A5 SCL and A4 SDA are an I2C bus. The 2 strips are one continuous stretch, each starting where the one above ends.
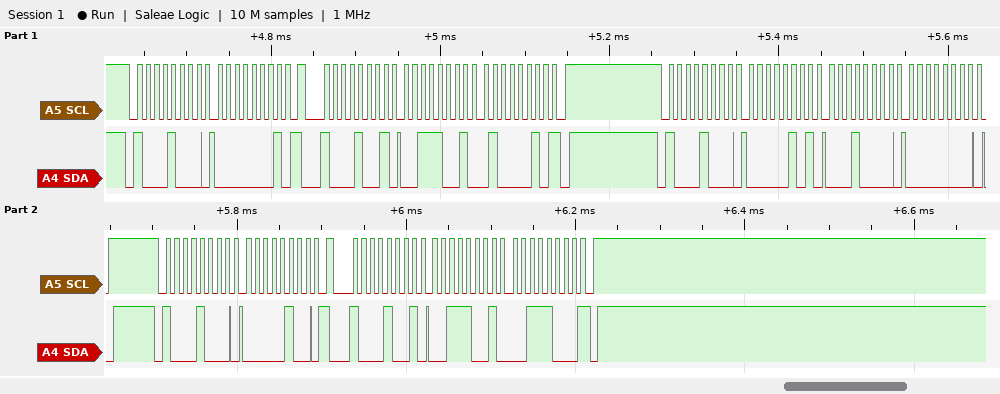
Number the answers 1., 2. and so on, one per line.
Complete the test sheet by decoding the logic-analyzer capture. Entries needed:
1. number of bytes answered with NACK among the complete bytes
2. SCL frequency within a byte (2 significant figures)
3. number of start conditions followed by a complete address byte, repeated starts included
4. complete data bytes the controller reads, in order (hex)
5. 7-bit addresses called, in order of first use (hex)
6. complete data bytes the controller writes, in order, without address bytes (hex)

1. 2
2. 100 kHz
3. 5
4. 39 42 39 38
5. 0x44
6. 01 05 10 00 04
